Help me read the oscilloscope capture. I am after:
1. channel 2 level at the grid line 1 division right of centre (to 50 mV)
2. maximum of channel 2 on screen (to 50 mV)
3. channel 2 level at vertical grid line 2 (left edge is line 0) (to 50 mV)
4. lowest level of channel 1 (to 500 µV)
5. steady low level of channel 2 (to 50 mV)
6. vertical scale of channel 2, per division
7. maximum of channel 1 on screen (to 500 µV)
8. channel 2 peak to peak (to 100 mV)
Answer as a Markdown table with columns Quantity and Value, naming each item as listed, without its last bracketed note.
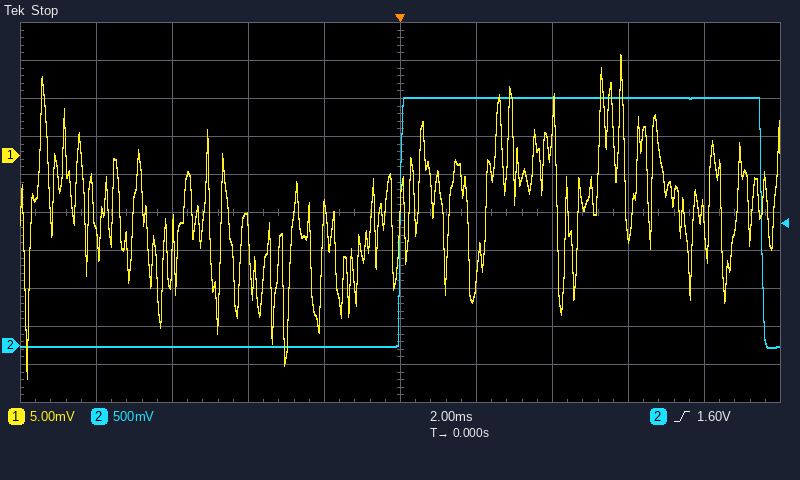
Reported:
| Quantity | Value |
|---|---|
| channel 2 level at the grid line 1 division right of centre | 3.25 V |
| maximum of channel 2 on screen | 3.25 V |
| channel 2 level at vertical grid line 2 (left edge is line 0) | 0 mV |
| lowest level of channel 1 | -29.5 mV |
| steady low level of channel 2 | 0 mV |
| vertical scale of channel 2, per division | 500 mV |
| maximum of channel 1 on screen | 13.5 mV |
| channel 2 peak to peak | 3.30 V |
